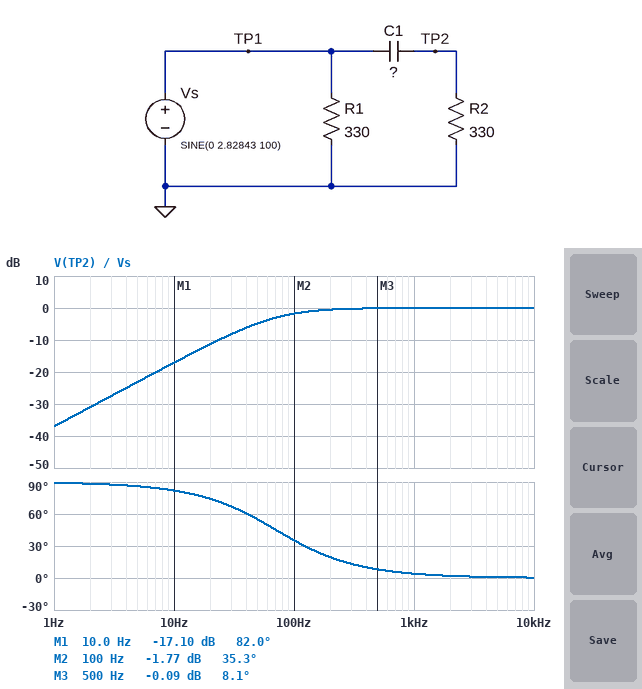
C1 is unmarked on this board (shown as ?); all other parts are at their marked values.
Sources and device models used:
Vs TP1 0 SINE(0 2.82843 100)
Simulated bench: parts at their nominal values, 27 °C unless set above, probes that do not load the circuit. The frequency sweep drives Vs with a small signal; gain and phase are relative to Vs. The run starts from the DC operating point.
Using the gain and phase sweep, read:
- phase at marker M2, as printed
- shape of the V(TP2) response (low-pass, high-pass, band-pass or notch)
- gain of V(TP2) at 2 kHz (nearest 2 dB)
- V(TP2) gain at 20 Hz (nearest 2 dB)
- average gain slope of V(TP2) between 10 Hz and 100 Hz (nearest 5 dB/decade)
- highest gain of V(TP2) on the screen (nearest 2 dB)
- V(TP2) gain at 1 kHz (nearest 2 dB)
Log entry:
35.3 deg
high-pass
0 dB
-12 dB
15 dB/decade
0 dB
0 dB
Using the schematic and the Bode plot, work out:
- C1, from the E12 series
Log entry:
6.8 µF
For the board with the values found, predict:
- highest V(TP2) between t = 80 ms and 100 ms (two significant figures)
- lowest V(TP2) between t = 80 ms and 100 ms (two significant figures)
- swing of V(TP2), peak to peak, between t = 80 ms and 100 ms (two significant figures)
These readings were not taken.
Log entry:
2.3 V
-2.3 V
4.6 V
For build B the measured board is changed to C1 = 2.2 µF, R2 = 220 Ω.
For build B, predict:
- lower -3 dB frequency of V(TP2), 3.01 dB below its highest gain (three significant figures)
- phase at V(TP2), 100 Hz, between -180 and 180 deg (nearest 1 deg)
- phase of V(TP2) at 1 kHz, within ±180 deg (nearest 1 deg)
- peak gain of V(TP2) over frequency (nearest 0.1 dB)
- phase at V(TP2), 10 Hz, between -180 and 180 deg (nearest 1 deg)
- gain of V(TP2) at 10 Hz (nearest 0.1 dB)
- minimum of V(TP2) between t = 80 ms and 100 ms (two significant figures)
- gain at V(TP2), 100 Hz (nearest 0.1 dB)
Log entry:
329 Hz
73 deg
18 deg
0 dB
88 deg
-30.3 dB
-820 mV
-10.7 dB
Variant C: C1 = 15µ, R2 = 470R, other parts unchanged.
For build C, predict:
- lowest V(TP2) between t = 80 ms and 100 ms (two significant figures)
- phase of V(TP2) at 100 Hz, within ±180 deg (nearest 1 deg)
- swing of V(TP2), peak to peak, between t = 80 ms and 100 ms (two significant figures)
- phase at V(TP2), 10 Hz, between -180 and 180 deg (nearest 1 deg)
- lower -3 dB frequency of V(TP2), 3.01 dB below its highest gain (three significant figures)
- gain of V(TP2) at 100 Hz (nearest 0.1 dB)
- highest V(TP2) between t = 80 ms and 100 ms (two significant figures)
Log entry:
-2.8 V
13 deg
5.5 V
66 deg
22.6 Hz
-0.2 dB
2.8 V
